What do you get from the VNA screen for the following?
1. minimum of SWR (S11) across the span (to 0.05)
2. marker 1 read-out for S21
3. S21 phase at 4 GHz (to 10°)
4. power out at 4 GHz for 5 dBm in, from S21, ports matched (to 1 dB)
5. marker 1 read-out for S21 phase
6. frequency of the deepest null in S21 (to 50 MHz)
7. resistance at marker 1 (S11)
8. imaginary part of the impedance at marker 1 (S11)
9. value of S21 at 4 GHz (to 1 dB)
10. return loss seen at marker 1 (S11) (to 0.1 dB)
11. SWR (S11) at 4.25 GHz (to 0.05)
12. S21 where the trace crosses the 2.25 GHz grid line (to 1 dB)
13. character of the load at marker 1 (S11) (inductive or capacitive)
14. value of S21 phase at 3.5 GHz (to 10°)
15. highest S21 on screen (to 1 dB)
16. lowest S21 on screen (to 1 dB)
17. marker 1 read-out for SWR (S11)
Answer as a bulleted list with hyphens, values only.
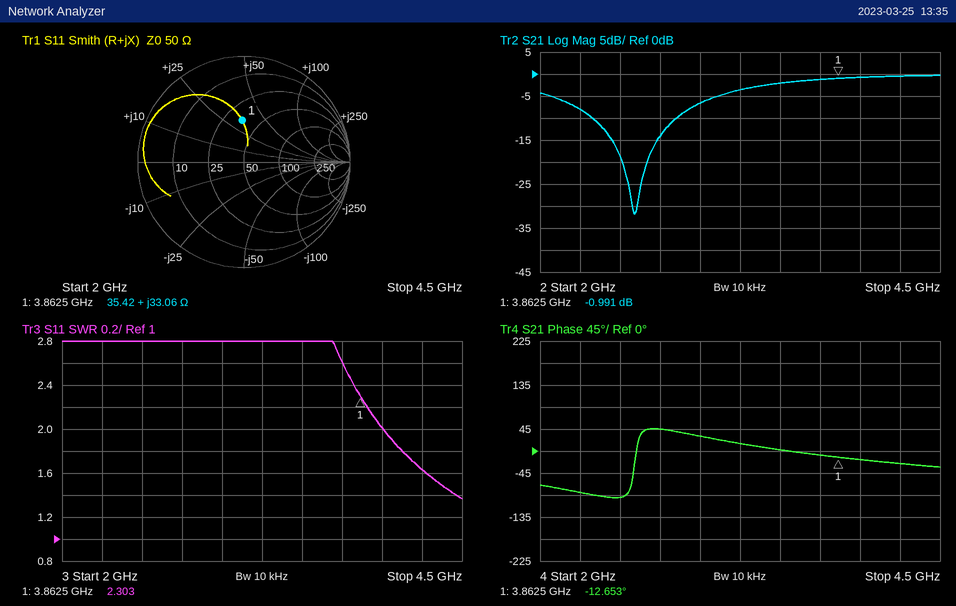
- 1.35
- -0.991 dB
- -20°
- 4 dBm
- -12.653°
- 2.60 GHz
- 35.42 Ω
- +33.06 Ω
- -1 dB
- 8.1 dB
- 1.65
- -8 dB
- inductive
- 0°
- 0 dB
- -32 dB
- 2.303
